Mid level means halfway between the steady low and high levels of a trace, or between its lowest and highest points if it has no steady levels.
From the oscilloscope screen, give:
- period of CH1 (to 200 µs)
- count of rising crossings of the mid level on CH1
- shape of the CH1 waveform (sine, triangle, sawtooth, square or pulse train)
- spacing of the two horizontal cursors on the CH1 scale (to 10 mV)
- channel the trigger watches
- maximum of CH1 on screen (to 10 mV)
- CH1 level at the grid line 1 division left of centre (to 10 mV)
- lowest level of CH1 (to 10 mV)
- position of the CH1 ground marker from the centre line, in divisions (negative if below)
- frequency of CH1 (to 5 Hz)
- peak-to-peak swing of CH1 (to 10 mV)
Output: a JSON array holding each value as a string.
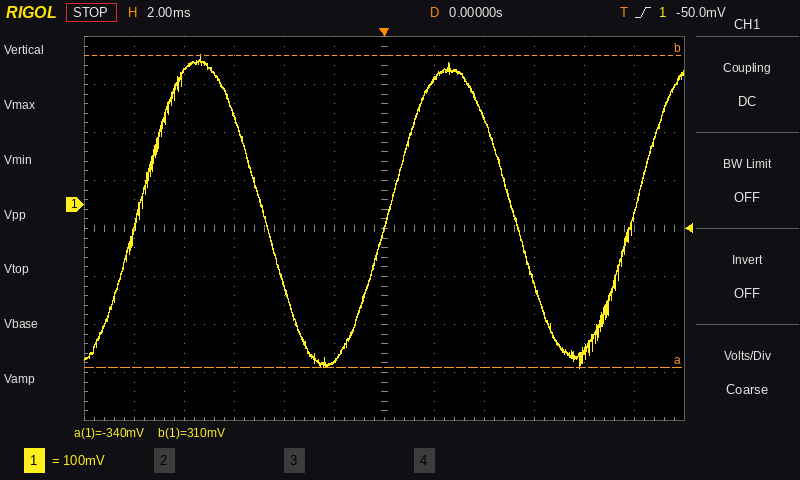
["10.0 ms", "3", "sine", "650 mV", "CH1", "310 mV", "-330 mV", "-340 mV", "+0.5 div", "100 Hz", "650 mV"]
